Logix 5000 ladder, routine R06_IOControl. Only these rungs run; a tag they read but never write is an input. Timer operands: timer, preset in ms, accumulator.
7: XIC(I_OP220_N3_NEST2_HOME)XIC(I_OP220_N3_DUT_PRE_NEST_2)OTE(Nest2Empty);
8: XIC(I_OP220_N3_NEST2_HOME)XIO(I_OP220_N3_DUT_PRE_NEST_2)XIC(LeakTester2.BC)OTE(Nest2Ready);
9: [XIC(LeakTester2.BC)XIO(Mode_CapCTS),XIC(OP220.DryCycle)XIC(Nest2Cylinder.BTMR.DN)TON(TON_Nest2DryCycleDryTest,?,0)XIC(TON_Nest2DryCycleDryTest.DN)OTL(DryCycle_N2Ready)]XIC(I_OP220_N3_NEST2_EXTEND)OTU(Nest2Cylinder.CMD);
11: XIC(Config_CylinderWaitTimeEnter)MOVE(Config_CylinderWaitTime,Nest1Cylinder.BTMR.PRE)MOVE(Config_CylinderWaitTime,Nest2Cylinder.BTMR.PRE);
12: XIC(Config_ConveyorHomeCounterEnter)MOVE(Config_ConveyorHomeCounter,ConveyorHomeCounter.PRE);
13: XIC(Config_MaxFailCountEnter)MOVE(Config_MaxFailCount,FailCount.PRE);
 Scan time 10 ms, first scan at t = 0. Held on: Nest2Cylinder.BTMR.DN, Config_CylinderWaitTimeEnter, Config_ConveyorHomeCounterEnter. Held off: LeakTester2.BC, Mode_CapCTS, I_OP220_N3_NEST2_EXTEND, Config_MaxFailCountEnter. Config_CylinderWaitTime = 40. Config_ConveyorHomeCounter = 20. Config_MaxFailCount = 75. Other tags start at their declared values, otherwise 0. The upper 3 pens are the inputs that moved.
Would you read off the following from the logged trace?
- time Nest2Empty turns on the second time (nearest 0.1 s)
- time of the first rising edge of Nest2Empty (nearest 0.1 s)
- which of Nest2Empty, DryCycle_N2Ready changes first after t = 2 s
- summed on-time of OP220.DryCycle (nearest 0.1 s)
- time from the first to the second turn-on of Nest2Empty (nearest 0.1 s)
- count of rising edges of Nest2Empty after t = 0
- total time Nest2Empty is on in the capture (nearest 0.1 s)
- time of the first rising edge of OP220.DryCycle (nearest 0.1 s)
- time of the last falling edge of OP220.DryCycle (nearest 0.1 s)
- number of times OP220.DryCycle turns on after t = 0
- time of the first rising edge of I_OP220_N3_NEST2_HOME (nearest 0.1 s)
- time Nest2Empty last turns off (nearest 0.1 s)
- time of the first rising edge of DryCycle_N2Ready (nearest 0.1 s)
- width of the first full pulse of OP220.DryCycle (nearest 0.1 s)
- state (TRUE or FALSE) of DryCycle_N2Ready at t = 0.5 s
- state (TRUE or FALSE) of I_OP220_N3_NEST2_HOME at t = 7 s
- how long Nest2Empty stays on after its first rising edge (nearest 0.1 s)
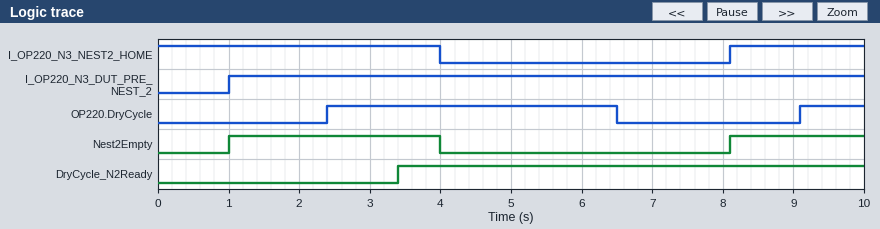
8.1 s
1.0 s
DryCycle_N2Ready
5.0 s
7.1 s
2
4.9 s
2.4 s
6.5 s
2
8.1 s
4.0 s
3.4 s
4.1 s
FALSE
FALSE
3.0 s
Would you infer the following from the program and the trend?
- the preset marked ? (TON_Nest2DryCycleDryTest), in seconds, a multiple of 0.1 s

1.0 s
